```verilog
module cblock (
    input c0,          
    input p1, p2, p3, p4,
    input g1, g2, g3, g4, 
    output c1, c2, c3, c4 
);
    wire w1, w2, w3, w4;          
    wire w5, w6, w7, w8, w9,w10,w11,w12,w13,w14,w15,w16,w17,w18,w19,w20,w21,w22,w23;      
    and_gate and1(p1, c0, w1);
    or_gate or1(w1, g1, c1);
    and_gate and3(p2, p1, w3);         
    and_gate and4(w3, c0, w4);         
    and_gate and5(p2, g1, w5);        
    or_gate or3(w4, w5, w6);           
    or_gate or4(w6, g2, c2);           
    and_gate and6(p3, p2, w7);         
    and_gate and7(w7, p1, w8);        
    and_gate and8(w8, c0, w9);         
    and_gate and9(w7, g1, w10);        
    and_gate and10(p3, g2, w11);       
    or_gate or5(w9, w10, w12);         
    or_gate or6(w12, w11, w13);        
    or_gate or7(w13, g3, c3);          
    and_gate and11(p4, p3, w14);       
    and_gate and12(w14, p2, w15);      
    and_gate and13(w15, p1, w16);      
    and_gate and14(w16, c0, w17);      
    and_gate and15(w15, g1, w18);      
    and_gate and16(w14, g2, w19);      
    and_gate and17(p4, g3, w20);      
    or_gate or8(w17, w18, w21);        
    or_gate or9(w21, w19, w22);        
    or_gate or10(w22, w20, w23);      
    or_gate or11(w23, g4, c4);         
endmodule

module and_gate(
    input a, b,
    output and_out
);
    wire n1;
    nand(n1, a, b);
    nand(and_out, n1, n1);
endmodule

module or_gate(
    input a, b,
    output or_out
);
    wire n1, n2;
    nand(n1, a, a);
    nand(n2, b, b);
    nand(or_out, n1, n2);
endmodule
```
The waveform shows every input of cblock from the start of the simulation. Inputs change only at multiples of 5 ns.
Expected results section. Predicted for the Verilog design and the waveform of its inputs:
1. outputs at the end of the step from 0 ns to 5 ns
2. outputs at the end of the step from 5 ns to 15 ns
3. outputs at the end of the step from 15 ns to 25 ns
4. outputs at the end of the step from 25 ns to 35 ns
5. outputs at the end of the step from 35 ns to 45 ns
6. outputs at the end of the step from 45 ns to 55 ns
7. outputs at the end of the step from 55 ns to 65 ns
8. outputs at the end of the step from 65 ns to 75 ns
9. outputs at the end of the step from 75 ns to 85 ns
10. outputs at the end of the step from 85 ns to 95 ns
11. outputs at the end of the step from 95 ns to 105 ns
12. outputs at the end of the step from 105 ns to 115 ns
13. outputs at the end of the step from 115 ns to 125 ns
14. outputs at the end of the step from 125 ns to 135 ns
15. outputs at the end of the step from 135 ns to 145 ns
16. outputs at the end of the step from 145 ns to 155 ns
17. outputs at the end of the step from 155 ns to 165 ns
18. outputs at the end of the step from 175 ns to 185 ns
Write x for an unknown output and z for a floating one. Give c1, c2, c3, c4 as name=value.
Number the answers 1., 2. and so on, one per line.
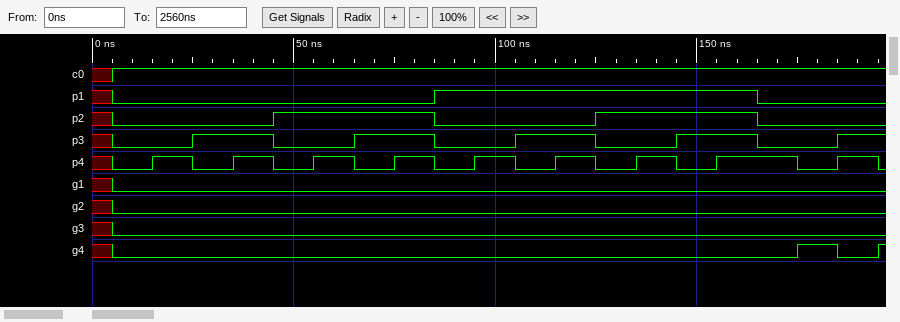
1. c1=x, c2=x, c3=x, c4=x
2. c1=0, c2=0, c3=0, c4=0
3. c1=0, c2=0, c3=0, c4=0
4. c1=0, c2=0, c3=0, c4=0
5. c1=0, c2=0, c3=0, c4=0
6. c1=0, c2=0, c3=0, c4=0
7. c1=0, c2=0, c3=0, c4=0
8. c1=0, c2=0, c3=0, c4=0
9. c1=0, c2=0, c3=0, c4=0
10. c1=1, c2=0, c3=0, c4=0
11. c1=1, c2=0, c3=0, c4=0
12. c1=1, c2=0, c3=0, c4=0
13. c1=1, c2=0, c3=0, c4=0
14. c1=1, c2=1, c3=0, c4=0
15. c1=1, c2=1, c3=0, c4=0
16. c1=1, c2=1, c3=1, c4=0
17. c1=1, c2=1, c3=1, c4=1
18. c1=0, c2=0, c3=0, c4=1
